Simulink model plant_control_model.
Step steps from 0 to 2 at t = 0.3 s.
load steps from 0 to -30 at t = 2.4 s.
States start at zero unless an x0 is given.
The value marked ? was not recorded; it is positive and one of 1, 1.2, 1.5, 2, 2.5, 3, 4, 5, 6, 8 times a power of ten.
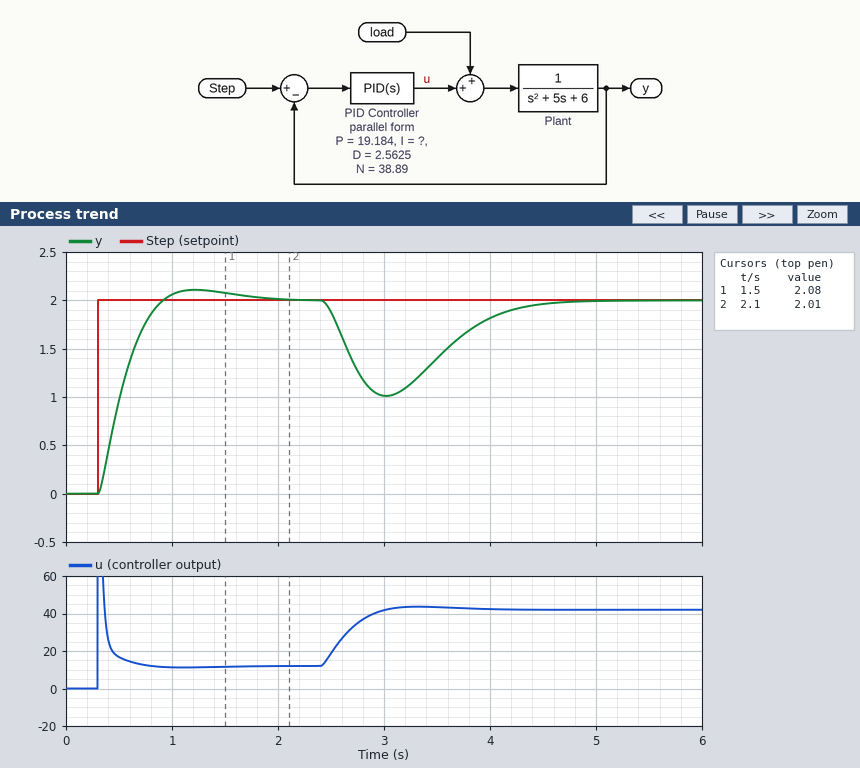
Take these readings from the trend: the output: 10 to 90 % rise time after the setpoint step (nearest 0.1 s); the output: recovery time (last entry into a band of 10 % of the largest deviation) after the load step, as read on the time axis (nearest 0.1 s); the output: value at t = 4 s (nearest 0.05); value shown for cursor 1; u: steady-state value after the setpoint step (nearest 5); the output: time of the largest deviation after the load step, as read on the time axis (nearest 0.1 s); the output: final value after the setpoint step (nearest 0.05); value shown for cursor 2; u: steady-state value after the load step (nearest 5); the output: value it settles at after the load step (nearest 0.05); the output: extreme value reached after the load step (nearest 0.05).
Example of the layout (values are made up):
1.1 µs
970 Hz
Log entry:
0.4 s
4.2 s
1.80
2.08
10
3.0 s
2.00
2.01
40
2.00
1.00
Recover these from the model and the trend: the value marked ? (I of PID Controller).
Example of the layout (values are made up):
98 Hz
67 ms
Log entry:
30
